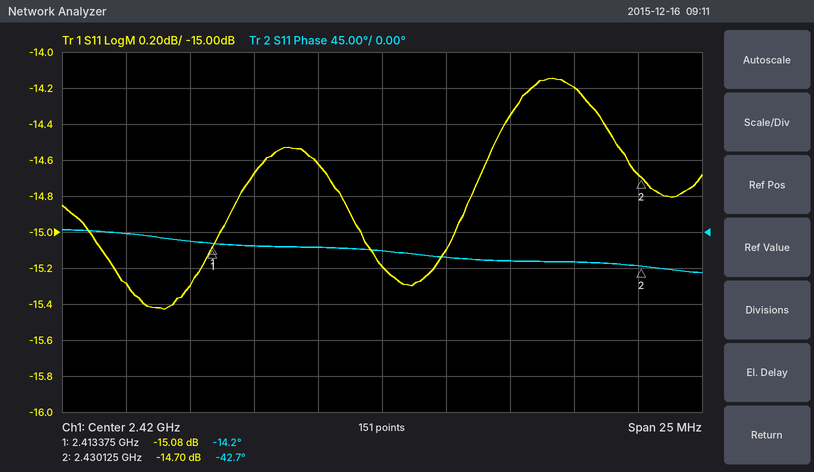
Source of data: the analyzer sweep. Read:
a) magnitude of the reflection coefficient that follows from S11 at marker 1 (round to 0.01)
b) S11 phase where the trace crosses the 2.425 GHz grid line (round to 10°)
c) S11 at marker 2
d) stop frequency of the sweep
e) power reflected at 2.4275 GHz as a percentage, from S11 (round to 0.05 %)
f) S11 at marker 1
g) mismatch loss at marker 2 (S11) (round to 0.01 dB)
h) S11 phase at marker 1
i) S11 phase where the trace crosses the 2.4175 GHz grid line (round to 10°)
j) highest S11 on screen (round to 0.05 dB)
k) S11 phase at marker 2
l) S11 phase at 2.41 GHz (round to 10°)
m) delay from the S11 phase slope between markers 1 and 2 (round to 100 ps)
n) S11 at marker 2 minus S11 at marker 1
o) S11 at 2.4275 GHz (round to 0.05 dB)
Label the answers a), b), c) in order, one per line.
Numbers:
a) 0.18
b) -40°
c) -14.70 dB
d) 2.4325 GHz
e) 3.80 %
f) -15.08 dB
g) 0.15 dB
h) -14.2°
i) -20°
j) -14.15 dB
k) -42.7°
l) 0°
m) 4.7 ns
n) 0.38 dB
o) -14.20 dB
